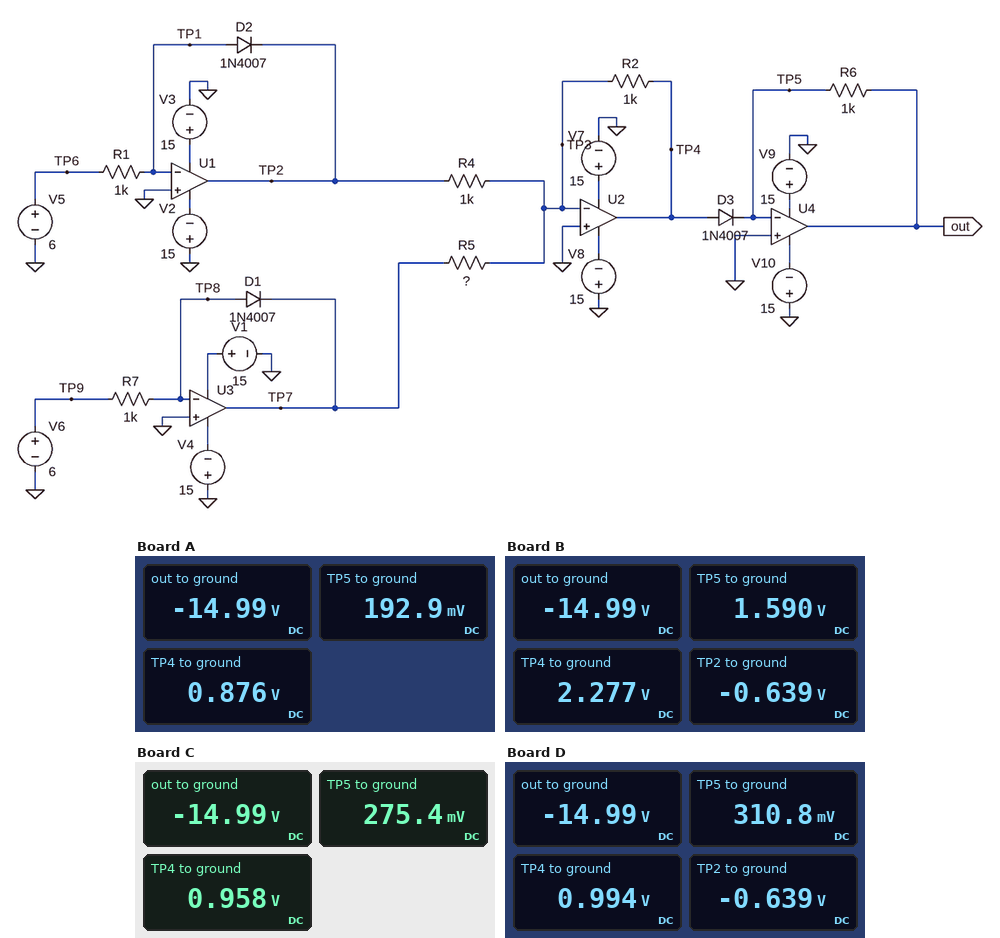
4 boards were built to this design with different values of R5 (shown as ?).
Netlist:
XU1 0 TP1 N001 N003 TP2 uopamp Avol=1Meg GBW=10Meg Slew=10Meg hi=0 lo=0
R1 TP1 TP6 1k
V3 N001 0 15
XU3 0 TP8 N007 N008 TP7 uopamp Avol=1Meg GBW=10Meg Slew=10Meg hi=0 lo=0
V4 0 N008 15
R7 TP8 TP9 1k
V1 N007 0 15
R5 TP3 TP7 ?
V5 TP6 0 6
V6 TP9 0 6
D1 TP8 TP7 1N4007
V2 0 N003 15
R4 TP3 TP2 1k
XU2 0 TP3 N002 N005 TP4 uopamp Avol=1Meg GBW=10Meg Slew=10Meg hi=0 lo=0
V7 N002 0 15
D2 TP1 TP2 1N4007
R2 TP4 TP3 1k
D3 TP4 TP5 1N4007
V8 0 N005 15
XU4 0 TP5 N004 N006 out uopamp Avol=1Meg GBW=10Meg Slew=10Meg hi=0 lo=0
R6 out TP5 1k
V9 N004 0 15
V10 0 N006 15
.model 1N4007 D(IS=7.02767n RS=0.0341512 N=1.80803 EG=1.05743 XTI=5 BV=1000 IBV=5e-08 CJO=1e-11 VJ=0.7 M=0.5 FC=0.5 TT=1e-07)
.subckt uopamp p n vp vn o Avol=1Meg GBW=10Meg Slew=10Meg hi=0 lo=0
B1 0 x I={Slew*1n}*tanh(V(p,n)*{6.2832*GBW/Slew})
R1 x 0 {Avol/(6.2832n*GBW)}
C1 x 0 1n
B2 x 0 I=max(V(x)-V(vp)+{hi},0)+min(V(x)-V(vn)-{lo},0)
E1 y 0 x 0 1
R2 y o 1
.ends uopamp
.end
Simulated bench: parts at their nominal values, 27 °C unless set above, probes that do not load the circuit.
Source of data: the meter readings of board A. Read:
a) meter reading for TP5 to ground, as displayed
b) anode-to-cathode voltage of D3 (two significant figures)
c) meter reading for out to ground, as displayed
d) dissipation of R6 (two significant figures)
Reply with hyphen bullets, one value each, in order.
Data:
- 192.9 mV
- 680 mV
- -14.99 V
- 230 mW
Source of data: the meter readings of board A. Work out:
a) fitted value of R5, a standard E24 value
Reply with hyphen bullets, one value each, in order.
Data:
- 2.7 kΩ
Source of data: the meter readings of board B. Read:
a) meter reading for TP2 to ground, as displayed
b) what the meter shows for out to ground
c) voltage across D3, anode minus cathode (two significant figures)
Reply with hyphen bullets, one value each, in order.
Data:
- -0.639 V
- -14.99 V
- 690 mV
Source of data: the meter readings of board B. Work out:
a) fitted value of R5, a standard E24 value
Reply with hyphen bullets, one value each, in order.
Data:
- 390 Ω
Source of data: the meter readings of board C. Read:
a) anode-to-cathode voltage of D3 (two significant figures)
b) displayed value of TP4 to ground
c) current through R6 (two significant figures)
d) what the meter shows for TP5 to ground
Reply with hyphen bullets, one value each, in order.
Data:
- 680 mV
- 0.958 V
- 15 mA
- 275.4 mV
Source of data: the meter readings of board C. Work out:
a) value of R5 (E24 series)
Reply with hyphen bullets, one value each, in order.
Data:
- 2 kΩ
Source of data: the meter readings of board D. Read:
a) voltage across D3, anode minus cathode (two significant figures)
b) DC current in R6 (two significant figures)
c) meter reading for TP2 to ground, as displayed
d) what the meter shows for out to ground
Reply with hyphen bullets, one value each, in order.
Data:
- 680 mV
- 15 mA
- -0.639 V
- -14.99 V
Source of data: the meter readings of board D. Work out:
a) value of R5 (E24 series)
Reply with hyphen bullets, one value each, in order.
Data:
- 1.8 kΩ
